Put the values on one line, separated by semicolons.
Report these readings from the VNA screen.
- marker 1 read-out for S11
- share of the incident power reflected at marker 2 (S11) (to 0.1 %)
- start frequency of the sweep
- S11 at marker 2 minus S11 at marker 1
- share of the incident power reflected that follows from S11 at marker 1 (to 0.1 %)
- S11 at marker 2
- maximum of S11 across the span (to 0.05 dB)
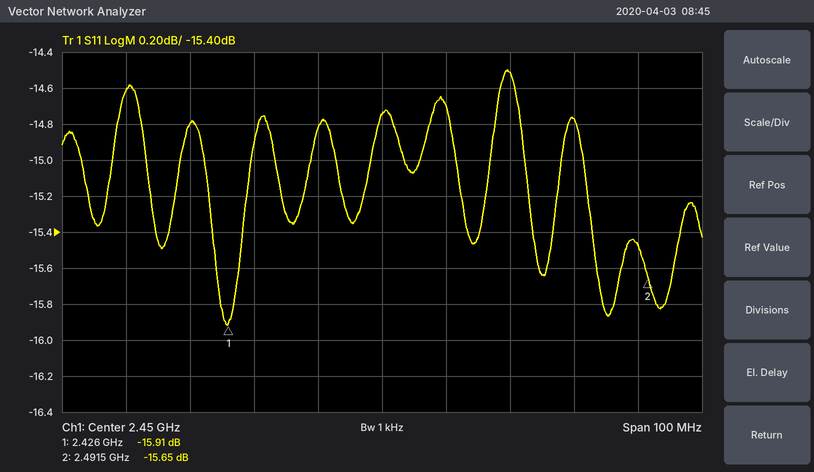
-15.91 dB; 2.7 %; 2.4 GHz; 0.26 dB; 2.6 %; -15.65 dB; -14.50 dB
